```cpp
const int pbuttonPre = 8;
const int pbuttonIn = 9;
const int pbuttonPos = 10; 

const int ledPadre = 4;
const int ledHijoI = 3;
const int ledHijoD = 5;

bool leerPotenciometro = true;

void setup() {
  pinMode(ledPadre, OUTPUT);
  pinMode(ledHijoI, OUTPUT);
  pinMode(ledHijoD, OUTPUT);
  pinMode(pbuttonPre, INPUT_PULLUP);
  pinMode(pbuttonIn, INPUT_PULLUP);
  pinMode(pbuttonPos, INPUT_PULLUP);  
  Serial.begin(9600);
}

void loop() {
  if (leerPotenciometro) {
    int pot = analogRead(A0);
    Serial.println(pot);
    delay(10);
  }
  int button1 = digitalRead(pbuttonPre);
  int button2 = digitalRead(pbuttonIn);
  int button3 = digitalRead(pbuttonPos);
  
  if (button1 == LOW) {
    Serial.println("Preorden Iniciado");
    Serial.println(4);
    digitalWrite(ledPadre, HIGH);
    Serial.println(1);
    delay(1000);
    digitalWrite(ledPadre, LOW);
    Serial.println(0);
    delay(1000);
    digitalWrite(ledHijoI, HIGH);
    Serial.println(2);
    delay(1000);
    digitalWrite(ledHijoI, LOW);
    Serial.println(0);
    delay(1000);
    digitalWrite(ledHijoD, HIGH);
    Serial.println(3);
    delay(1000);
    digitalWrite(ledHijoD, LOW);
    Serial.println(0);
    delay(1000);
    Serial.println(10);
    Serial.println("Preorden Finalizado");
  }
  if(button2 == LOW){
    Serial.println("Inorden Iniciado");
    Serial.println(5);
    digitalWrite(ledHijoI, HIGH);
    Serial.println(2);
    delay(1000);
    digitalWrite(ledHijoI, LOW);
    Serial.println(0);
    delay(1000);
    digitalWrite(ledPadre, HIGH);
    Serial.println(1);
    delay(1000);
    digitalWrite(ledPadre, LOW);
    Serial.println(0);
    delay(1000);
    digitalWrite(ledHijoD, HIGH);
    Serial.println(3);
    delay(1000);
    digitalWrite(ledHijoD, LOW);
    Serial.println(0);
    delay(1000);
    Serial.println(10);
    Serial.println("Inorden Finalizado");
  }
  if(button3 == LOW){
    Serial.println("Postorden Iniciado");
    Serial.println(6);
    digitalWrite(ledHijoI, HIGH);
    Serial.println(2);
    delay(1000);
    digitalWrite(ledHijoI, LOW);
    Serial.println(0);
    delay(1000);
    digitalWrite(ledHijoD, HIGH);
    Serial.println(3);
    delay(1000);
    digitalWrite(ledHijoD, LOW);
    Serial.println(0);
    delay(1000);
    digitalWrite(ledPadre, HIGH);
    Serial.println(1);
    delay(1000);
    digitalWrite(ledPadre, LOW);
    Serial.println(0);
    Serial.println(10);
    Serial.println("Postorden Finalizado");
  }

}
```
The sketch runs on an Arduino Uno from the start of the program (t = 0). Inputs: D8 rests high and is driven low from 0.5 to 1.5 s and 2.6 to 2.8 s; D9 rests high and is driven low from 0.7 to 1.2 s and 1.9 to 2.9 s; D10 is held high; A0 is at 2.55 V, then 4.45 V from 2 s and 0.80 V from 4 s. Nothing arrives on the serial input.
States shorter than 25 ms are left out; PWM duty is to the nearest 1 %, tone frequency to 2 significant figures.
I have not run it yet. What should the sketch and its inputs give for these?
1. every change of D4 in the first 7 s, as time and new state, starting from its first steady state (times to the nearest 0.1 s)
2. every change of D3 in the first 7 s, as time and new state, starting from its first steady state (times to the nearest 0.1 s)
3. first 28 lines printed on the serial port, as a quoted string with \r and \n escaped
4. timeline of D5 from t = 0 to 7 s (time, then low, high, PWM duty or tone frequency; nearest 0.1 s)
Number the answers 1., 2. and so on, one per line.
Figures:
1. 0 s low; 0.5 s high; 1.5 s low
2. 0 s low; 2.5 s high; 3.5 s low
3. "522\r\n522\r\n522\r\n522\r\n522\r\n522\r\n522\r\n522\r\n522\r\n522\r\n522\r\n522\r\n522\r\n522\r\n522\r\n522\r\n522\r\n522\r\n522\r\n522\r\n522\r\n522\r\n522\r\n522\r\n522\r\n522\r\n522\r\n522\r\n"
4. 0 s low; 4.5 s high; 5.5 s low
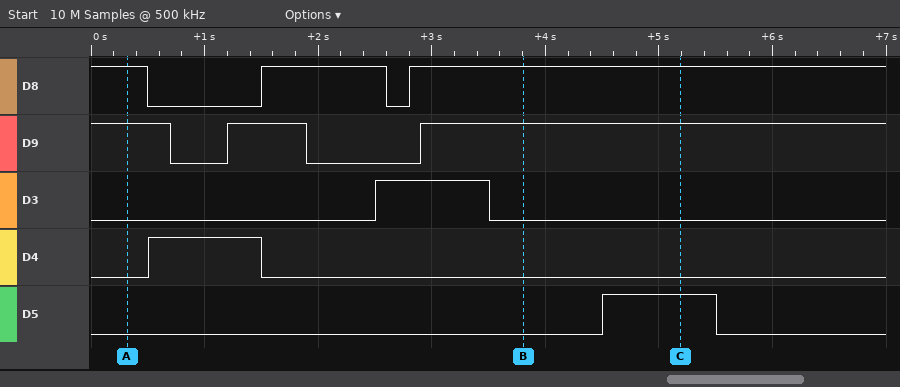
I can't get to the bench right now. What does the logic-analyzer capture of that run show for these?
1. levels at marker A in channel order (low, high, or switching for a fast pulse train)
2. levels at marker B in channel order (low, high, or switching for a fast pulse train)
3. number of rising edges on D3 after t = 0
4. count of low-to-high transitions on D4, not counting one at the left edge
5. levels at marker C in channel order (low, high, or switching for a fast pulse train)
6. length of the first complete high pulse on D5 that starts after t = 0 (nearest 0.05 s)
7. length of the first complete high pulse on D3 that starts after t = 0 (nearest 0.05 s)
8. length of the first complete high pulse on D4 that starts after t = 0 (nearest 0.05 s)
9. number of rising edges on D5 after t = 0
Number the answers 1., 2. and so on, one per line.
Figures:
1. D8 high, D9 high, D3 low, D4 low, D5 low
2. D8 high, D9 high, D3 low, D4 low, D5 low
3. 1
4. 1
5. D8 high, D9 high, D3 low, D4 low, D5 high
6. 1.00 s
7. 1.00 s
8. 1.00 s
9. 1
